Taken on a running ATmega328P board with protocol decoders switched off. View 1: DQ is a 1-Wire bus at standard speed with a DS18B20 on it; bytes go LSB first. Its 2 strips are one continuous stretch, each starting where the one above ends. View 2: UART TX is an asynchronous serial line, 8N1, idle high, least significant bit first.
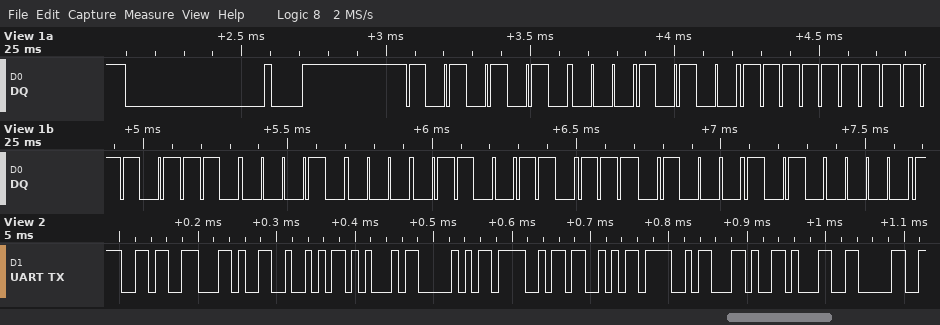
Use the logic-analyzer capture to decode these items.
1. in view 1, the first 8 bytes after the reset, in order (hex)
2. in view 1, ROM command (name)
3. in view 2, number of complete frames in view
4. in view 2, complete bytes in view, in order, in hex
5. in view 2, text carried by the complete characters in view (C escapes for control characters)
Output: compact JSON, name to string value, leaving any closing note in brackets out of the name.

{"in view 1, the first 8 bytes after the reset, in order": "55 28 FF 77 08 66 17 05", "in view 1, ROM command": "Match ROM", "in view 2, number of complete frames in view": "11", "in view 2, complete bytes in view, in order, in hex": "0x36 0x2C 0x52 0x45 0x50 0x4F 0x53 0x4F 0x2C 0x31 0x30", "in view 2, text carried by the complete characters in view": "\"6,REPOSO,10\""}
